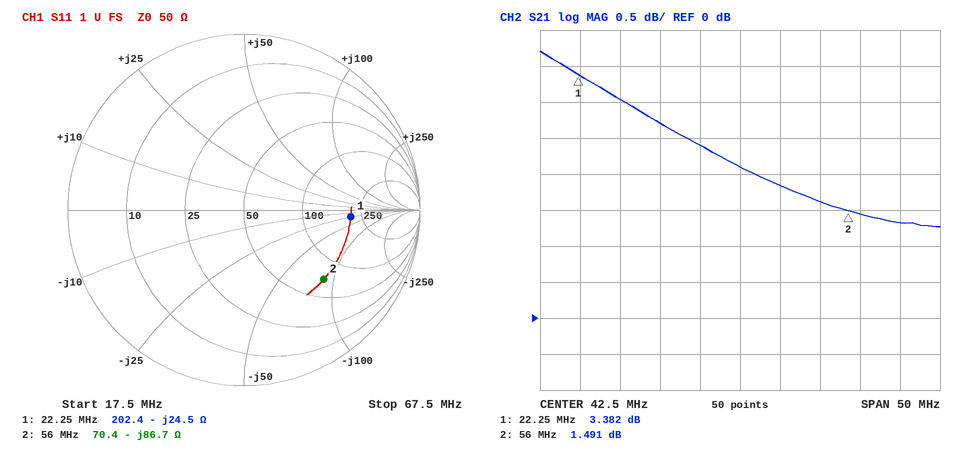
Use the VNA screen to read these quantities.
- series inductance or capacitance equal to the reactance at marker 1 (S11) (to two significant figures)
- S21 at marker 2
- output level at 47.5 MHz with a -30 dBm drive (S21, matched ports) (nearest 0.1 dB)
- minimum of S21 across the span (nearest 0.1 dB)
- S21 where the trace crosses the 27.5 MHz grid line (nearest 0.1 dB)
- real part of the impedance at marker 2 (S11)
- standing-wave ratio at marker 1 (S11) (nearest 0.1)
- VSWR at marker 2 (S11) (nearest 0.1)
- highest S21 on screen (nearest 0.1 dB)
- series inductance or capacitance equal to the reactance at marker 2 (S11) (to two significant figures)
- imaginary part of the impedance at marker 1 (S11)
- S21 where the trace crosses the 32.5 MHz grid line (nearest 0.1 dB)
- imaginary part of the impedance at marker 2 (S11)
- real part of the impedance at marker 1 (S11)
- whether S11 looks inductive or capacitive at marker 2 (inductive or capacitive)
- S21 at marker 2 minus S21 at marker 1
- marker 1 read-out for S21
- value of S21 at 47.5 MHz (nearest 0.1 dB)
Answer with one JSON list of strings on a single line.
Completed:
["290 pF", "1.491 dB", "-28.2 dBm", "1.3 dB", "3.0 dB", "70.4 Ω", "4.1", "4.0", "3.7 dB", "33 pF", "-24.5 Ω", "2.7 dB", "-86.7 Ω", "202.4 Ω", "capacitive", "-1.891 dB", "3.382 dB", "1.8 dB"]
